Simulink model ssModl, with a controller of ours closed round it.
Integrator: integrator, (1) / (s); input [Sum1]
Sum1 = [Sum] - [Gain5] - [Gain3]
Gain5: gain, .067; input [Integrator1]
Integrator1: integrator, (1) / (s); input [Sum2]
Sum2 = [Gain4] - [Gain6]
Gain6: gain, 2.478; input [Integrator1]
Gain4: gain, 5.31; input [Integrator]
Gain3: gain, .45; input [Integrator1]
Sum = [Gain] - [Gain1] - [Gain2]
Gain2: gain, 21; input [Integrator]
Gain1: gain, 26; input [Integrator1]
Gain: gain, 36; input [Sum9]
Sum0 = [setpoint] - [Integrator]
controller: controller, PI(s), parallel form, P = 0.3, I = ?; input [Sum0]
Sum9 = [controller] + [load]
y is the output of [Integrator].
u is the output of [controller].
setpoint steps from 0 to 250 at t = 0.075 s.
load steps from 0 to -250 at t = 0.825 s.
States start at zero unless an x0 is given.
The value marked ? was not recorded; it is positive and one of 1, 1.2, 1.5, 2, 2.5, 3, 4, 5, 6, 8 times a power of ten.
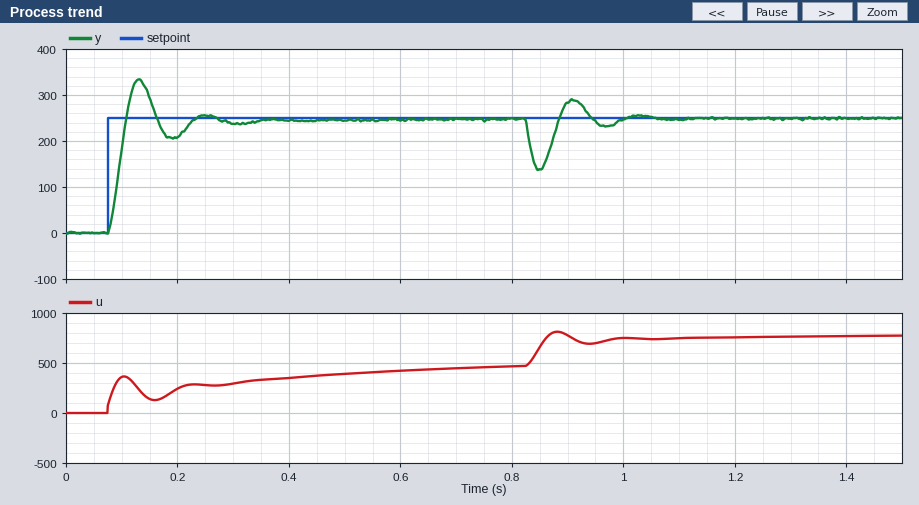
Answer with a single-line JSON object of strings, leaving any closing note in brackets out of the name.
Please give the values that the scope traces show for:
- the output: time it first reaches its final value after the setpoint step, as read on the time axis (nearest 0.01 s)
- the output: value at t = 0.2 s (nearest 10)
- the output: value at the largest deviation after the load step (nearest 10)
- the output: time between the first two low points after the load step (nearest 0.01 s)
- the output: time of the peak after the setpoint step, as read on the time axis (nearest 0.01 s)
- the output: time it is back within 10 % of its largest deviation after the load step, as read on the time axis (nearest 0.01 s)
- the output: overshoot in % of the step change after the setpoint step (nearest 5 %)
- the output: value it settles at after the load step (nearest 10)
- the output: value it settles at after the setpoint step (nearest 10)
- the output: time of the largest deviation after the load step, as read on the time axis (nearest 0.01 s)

{"the output: time it first reaches its final value after the setpoint step, as read on the time axis": "0.11 s", "the output: value at t = 0.2 s": "210", "the output: value at the largest deviation after the load step": "140", "the output: time between the first two low points after the load step": "0.12 s", "the output: time of the peak after the setpoint step, as read on the time axis": "0.13 s", "the output: time it is back within 10 % of its largest deviation after the load step, as read on the time axis": "0.99 s", "the output: overshoot in % of the step change after the setpoint step": "35 %", "the output: value it settles at after the load step": "250", "the output: value it settles at after the setpoint step": "250", "the output: time of the largest deviation after the load step, as read on the time axis": "0.85 s"}
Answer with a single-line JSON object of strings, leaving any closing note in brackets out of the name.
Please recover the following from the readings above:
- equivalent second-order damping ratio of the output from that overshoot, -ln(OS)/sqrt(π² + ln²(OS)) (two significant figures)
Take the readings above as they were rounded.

{"equivalent second-order damping ratio of the output from that overshoot, -ln(OS)/sqrt(π² + ln²(OS))": "0.32"}
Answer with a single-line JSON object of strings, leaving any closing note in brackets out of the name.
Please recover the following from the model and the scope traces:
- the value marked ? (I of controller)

{"the value marked ?": "80"}
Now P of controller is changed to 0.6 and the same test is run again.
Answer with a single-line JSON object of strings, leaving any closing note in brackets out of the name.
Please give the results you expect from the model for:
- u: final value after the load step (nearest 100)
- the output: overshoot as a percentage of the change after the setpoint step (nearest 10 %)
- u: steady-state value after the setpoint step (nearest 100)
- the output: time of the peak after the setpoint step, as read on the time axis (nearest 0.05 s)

{"u: final value after the load step": "800", "the output: overshoot as a percentage of the change after the setpoint step": "20 %", "u: steady-state value after the setpoint step": "500", "the output: time of the peak after the setpoint step, as read on the time axis": "0.15 s"}
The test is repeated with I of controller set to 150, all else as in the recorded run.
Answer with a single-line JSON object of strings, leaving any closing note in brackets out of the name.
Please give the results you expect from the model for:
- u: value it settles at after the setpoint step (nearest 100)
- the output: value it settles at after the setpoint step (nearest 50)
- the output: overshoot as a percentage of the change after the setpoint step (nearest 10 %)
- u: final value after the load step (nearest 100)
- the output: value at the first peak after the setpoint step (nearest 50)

{"u: value it settles at after the setpoint step": "500", "the output: value it settles at after the setpoint step": "250", "the output: overshoot as a percentage of the change after the setpoint step": "50 %", "u: final value after the load step": "800", "the output: value at the first peak after the setpoint step": "350"}
